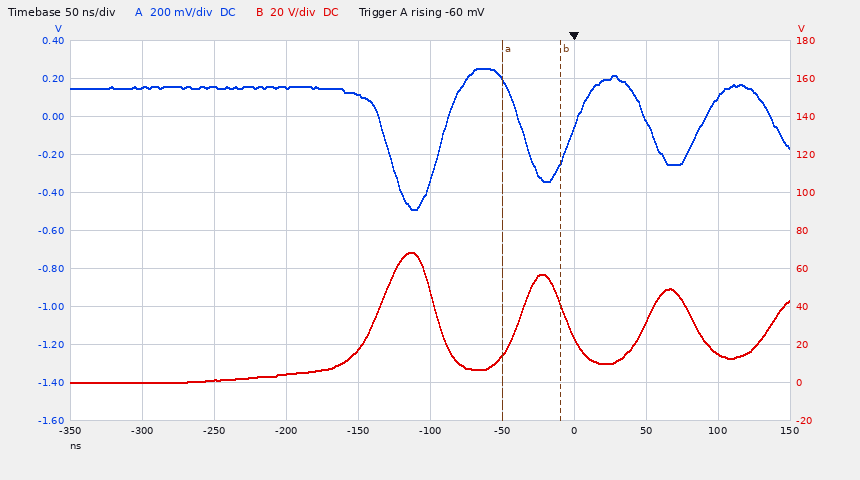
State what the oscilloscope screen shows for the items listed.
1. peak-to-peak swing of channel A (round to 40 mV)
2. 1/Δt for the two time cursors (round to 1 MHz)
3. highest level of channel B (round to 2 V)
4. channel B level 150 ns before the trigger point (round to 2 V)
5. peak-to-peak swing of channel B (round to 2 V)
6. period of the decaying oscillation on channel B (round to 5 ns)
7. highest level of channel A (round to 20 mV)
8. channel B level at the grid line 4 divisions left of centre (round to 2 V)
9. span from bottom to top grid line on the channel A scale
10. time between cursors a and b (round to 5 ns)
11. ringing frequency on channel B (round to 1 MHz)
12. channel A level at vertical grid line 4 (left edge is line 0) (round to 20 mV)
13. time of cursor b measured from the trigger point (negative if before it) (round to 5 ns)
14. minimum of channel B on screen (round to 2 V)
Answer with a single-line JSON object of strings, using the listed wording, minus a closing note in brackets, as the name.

{"peak-to-peak swing of channel A": "760 mV", "1/Δt for the two time cursors": "25 MHz", "highest level of channel B": "68 V", "channel B level 150 ns before the trigger point": "18 V", "peak-to-peak swing of channel B": "68 V", "period of the decaying oscillation on channel B": "90 ns", "highest level of channel A": "260 mV", "channel B level at the grid line 4 divisions left of centre": "0 V", "span from bottom to top grid line on the channel A scale": "2 V", "time between cursors a and b": "40 ns", "ringing frequency on channel B": "11 MHz", "channel A level at vertical grid line 4 (left edge is line 0)": "120 mV", "time of cursor b measured from the trigger point (negative if before it)": "-10 ns", "minimum of channel B on screen": "0 V"}
